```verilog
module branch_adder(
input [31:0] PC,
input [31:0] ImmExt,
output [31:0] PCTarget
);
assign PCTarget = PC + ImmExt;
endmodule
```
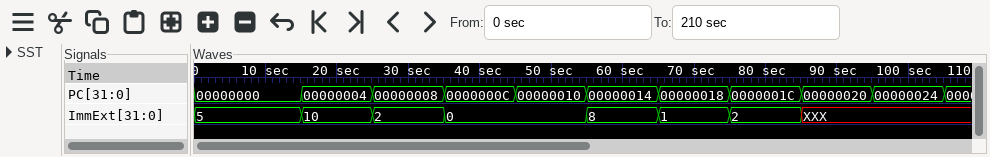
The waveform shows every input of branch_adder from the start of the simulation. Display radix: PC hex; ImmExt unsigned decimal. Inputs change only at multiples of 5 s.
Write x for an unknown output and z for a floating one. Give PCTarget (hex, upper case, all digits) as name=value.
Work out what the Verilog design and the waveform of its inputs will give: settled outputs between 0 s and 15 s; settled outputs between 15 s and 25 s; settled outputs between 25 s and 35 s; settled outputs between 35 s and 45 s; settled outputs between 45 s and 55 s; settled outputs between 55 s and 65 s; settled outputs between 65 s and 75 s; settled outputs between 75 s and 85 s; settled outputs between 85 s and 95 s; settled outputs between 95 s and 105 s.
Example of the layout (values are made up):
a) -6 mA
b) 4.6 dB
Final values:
a) PCTarget=00000005
b) PCTarget=0000000E
c) PCTarget=0000000A
d) PCTarget=0000000C
e) PCTarget=00000010
f) PCTarget=0000001C
g) PCTarget=00000019
h) PCTarget=0000001E
i) PCTarget=x
j) PCTarget=x
